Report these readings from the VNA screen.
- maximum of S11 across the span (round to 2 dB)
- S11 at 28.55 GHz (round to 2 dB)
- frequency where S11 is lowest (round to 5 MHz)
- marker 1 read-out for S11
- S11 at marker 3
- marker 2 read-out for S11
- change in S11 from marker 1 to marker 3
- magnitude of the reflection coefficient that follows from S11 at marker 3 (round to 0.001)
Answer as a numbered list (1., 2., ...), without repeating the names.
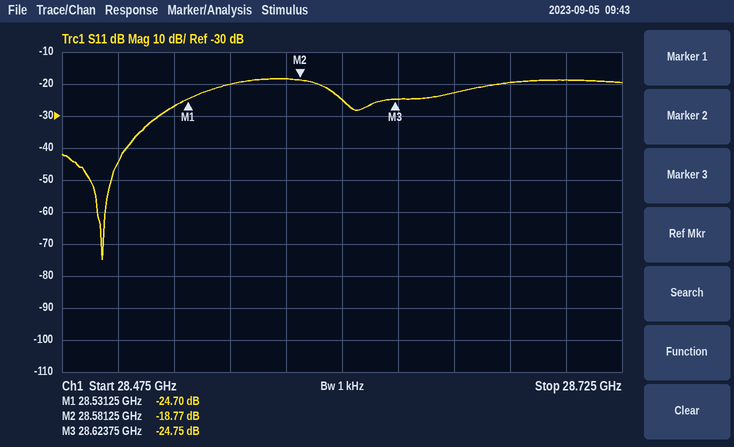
1. -18 dB
2. -20 dB
3. 28.495 GHz
4. -24.70 dB
5. -24.75 dB
6. -18.77 dB
7. -0.05 dB
8. 0.058
